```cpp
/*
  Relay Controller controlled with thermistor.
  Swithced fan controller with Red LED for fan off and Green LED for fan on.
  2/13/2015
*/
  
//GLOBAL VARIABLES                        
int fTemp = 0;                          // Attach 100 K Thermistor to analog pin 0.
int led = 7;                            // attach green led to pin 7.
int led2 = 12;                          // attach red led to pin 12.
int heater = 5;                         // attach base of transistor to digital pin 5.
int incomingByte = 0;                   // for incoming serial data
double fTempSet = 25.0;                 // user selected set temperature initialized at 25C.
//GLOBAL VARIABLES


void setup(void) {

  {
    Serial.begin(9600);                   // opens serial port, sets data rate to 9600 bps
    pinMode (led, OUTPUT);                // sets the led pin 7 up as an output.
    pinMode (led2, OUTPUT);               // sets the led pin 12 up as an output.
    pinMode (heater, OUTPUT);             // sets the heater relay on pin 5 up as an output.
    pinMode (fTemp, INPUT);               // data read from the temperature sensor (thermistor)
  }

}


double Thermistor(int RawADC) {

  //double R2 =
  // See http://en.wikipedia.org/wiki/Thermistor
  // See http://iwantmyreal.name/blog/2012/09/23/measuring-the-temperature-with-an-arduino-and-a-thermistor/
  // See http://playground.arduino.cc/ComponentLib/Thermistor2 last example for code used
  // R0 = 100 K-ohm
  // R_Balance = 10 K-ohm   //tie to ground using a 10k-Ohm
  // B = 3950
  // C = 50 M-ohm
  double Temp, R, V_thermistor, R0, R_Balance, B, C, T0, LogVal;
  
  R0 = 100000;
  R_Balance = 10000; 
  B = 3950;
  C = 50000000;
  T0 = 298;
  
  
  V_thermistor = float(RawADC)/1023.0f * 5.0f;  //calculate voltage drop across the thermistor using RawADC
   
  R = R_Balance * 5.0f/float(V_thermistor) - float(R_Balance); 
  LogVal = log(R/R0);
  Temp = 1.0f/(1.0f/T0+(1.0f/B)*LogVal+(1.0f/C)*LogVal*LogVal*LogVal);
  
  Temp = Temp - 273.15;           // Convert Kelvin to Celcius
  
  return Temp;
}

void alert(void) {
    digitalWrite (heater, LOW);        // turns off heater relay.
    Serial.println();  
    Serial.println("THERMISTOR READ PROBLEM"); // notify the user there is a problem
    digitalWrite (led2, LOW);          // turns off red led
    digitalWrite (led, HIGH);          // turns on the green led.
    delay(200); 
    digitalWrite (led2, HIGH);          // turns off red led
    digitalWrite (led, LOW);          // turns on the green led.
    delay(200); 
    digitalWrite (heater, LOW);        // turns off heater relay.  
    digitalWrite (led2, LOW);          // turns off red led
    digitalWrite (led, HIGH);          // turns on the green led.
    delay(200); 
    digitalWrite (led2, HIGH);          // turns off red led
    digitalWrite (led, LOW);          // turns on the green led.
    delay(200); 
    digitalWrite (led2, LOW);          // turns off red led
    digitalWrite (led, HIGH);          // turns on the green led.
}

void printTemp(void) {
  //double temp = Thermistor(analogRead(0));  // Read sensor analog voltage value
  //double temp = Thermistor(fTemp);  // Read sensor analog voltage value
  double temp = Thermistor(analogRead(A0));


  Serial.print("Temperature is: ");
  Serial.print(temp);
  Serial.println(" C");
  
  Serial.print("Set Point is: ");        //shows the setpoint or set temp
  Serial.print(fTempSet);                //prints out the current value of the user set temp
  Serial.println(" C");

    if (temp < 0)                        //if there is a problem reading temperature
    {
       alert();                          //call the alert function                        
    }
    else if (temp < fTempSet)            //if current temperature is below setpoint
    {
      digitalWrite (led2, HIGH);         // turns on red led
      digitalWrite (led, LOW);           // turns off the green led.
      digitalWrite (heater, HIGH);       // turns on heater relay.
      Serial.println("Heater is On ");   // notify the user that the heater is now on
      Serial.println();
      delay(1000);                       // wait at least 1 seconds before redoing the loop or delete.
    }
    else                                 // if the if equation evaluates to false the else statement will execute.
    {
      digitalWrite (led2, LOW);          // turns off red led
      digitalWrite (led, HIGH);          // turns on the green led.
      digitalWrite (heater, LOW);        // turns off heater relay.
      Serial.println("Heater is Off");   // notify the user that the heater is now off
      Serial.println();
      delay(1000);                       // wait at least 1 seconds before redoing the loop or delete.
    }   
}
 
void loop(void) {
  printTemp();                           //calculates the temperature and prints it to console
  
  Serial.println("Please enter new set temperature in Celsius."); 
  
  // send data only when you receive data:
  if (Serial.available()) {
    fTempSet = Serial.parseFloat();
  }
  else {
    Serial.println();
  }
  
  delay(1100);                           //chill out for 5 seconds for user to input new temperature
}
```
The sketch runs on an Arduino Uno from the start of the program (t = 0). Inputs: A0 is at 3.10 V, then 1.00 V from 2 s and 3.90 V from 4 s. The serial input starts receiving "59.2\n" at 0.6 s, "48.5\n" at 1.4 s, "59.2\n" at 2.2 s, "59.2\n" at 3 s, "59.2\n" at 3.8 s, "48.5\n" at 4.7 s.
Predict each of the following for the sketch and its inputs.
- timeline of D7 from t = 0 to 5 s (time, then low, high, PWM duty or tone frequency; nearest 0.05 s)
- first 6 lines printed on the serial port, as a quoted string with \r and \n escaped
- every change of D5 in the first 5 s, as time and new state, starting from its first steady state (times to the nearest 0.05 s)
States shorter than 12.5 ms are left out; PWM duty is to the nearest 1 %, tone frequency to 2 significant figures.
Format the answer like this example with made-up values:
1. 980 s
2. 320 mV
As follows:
1. 0 s high; 2.1 s low; 4.2 s high
2. "Temperature is: 104.40 C\r\nSet Point is: 25.00 C\r\nHeater is Off\r\n\r\nPlease enter new set temperature in Celsius.\r\nTemperature is: 46.89 C\r\n"
3. 0 s low; 2.1 s high; 4.2 s low
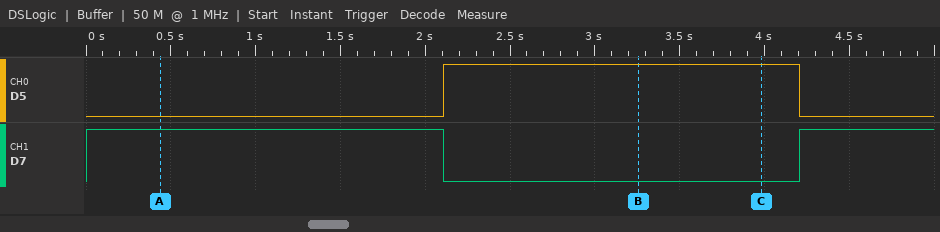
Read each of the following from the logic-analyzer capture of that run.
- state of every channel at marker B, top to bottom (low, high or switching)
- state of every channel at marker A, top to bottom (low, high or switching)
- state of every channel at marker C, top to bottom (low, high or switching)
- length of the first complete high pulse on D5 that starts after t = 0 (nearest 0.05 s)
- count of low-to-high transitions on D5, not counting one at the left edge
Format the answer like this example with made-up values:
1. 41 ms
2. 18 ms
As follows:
1. D5 high, D7 low
2. D5 low, D7 high
3. D5 high, D7 low
4. 2.10 s
5. 1
